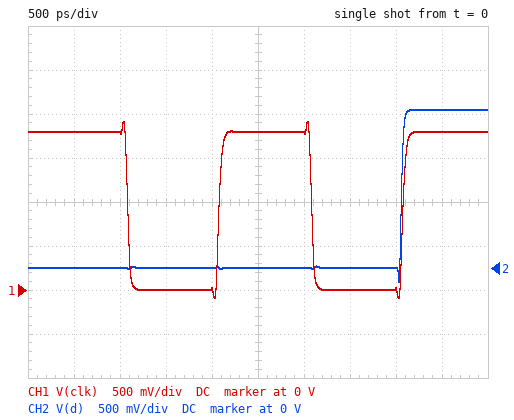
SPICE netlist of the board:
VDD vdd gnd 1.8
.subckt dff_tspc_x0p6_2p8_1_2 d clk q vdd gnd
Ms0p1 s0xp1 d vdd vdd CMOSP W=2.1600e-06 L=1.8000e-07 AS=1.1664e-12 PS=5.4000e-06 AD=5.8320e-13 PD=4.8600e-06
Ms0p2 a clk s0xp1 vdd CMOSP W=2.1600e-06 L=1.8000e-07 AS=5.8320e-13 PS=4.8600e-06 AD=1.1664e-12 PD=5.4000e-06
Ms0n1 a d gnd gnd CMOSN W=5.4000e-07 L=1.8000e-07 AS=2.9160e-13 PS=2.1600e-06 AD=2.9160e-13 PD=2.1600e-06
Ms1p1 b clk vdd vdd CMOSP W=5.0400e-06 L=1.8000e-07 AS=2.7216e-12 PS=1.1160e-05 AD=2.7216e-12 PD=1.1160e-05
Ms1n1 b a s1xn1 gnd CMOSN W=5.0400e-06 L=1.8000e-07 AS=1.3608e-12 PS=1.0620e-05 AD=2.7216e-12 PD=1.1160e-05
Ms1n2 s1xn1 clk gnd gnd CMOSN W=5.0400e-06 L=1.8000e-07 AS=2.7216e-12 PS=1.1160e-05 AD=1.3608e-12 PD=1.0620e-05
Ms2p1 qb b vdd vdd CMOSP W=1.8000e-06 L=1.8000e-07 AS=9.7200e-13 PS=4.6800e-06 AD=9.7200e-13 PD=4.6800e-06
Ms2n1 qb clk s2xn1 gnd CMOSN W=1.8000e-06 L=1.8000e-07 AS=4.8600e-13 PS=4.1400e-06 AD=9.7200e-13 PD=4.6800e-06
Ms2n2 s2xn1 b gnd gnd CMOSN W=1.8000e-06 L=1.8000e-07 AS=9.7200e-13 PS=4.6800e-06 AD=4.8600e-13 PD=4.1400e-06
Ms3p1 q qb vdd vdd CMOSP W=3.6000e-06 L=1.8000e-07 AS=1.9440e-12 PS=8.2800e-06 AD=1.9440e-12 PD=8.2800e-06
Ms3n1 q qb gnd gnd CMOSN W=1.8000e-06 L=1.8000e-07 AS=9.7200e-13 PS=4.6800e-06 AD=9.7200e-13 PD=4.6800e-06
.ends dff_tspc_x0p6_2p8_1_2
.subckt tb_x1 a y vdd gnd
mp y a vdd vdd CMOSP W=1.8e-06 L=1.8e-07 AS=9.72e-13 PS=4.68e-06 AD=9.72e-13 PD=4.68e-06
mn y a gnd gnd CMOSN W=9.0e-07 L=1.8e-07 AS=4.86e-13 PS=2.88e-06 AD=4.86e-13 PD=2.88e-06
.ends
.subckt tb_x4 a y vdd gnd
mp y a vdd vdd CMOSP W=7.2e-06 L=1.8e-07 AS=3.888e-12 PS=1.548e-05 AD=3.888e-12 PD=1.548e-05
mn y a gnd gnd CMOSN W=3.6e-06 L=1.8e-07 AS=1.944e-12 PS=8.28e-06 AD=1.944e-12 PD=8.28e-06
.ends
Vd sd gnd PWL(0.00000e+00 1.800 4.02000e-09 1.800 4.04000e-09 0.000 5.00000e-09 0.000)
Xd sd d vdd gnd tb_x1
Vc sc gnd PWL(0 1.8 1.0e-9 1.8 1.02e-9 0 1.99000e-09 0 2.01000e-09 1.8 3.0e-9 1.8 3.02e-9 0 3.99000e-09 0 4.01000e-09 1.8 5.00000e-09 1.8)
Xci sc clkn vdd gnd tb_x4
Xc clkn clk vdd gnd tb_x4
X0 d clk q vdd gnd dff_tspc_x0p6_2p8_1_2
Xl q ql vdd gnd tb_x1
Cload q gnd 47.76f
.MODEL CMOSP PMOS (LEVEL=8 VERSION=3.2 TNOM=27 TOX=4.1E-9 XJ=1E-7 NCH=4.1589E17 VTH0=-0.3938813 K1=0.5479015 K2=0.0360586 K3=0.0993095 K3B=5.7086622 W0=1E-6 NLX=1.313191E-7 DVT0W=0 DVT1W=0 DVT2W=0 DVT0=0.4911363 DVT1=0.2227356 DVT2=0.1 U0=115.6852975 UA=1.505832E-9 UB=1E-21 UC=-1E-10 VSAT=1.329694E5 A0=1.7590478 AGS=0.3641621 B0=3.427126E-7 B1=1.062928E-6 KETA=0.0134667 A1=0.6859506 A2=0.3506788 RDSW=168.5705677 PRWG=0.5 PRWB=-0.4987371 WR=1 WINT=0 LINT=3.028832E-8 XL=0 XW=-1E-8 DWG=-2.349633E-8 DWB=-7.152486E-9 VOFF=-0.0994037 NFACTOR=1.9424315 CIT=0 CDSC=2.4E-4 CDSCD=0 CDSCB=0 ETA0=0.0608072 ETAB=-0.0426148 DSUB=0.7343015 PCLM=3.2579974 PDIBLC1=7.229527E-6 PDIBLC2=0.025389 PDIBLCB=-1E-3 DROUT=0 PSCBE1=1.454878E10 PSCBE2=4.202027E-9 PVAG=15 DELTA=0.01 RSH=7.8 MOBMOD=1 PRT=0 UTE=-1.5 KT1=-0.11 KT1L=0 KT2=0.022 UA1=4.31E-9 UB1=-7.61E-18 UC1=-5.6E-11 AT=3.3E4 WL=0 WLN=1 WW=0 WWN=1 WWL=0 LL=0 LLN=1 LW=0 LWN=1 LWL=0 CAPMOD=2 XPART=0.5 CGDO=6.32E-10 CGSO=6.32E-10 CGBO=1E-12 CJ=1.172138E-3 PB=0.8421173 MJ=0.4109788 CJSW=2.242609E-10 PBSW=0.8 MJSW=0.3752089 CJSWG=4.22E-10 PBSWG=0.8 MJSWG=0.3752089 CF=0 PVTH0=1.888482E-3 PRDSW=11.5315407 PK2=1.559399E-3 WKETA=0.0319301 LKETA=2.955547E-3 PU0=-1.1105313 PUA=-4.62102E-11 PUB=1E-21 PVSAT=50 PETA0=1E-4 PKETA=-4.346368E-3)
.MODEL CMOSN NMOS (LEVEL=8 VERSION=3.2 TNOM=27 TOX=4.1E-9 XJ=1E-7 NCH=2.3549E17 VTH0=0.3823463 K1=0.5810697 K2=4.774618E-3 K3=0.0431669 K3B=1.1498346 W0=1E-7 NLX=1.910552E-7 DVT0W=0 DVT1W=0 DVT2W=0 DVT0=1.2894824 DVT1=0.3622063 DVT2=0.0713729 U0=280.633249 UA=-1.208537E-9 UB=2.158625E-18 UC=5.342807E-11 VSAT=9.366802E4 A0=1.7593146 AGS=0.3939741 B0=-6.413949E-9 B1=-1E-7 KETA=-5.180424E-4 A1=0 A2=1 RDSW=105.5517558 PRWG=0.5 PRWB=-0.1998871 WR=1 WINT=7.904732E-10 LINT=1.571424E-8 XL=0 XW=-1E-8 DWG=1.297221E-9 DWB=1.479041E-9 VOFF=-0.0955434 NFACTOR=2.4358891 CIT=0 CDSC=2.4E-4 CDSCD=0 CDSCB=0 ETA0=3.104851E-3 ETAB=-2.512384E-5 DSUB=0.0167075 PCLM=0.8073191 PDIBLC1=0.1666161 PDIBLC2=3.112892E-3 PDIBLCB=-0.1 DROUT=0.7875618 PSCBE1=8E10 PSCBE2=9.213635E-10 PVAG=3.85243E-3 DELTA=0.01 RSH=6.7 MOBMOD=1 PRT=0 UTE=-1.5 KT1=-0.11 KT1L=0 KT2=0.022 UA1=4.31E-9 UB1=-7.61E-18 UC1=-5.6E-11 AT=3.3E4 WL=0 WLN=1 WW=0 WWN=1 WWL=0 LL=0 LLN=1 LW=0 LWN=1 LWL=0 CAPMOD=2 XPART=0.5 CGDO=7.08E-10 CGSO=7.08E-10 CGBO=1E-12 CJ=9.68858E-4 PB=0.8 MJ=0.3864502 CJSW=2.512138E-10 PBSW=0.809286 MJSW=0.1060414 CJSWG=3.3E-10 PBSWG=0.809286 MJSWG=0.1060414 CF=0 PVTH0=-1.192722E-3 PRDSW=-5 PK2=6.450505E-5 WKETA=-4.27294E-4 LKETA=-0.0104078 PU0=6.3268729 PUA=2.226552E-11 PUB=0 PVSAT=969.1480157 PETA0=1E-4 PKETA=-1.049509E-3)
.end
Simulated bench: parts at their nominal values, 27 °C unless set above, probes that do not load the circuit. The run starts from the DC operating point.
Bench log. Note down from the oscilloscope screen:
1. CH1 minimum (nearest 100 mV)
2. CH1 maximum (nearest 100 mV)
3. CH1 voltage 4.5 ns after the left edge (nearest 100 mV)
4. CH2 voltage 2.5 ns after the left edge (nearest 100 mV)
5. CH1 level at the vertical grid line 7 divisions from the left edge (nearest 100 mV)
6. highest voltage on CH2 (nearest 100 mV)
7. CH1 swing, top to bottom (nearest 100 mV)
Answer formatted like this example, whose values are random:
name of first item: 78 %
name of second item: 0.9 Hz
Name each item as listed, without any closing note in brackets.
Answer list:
CH1 minimum: -100 mV
CH1 maximum: 1.9 V
CH1 voltage 4.5 ns after the left edge: 1.8 V
CH2 voltage 2.5 ns after the left edge: 0 V
CH1 level at the vertical grid line 7 divisions from the left edge: 0 V
highest voltage on CH2: 1.8 V
CH1 swing, top to bottom: 2.0 V
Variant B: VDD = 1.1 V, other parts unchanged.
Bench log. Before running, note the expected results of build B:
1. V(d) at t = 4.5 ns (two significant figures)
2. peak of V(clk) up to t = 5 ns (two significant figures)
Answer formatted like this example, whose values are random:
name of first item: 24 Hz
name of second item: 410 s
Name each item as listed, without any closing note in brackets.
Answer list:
V(d) at t = 4.5 ns: 1.1 V
peak of V(clk) up to t = 5 ns: 1.2 V
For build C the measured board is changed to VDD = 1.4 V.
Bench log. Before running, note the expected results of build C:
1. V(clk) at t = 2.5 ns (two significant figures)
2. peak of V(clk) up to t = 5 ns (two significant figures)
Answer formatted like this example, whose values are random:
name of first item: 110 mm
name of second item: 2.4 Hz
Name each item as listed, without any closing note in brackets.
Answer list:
V(clk) at t = 2.5 ns: 1.4 V
peak of V(clk) up to t = 5 ns: 1.5 V
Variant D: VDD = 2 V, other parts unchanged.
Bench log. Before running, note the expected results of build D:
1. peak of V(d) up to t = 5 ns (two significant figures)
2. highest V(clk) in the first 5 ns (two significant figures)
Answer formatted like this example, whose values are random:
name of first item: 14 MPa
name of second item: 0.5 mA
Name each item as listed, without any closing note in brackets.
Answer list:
peak of V(d) up to t = 5 ns: 2.0 V
highest V(clk) in the first 5 ns: 2.1 V
